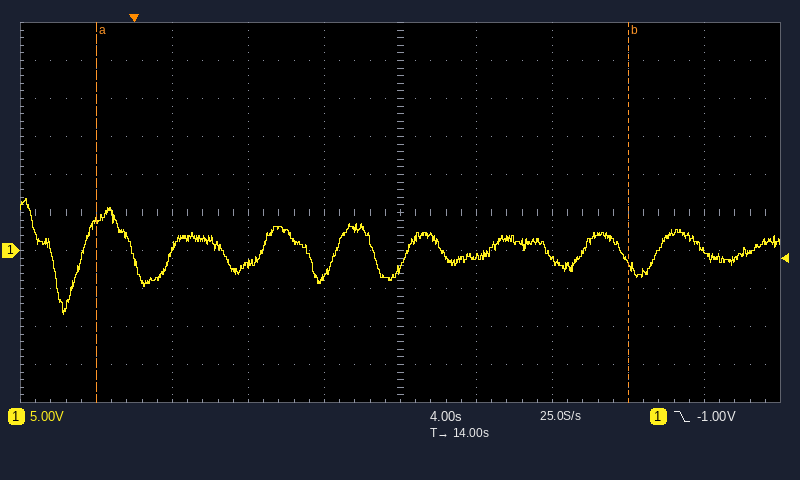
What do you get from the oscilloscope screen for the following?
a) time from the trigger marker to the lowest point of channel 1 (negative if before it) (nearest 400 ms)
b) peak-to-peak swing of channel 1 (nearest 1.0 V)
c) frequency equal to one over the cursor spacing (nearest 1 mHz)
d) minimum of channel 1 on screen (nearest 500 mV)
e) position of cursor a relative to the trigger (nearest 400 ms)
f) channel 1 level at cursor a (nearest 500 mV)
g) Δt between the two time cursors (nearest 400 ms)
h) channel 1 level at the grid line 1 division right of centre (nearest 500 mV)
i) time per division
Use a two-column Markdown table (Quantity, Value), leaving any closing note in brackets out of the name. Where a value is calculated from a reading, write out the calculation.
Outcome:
| Quantity | Value |
|---|---|
| time from the trigger marker to the lowest point of channel 1 (negative if before it) | -3.6 s |
| peak-to-peak swing of channel 1 | 15.0 V |
| frequency equal to one over the cursor spacing | 1 / 28.0 s ≈ 36 mHz |
| minimum of channel 1 on screen | -8.5 V |
| position of cursor a relative to the trigger | -2.0 s |
| channel 1 level at cursor a | 4.0 V |
| Δt between the two time cursors | 28.0 s |
| channel 1 level at the grid line 1 division right of centre | -1.0 V |
| time per division | 4 s |
